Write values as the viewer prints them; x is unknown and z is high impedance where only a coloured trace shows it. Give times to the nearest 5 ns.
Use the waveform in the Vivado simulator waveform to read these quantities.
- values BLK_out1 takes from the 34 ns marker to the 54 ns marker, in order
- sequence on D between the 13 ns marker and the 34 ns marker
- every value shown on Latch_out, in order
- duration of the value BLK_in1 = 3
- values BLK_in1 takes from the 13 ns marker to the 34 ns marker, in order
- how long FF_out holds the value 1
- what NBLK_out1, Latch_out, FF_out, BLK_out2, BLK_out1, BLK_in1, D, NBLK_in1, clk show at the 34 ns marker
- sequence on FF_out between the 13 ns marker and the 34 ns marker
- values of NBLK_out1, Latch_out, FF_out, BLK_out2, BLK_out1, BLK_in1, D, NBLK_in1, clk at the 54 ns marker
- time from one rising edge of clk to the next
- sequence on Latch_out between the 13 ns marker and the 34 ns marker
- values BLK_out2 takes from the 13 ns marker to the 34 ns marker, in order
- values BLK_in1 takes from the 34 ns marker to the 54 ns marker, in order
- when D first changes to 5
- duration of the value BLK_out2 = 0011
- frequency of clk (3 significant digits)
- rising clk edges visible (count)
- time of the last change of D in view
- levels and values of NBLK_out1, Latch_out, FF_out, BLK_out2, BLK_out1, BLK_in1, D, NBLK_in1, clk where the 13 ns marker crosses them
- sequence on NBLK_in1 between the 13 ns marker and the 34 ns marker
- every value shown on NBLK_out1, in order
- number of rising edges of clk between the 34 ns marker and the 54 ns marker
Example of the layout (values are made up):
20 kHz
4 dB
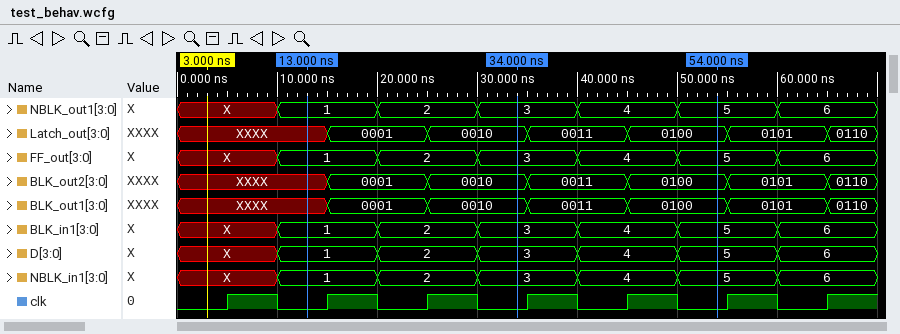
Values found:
0010, 0011, 0100
1, 2, 3
XXXX, 0001, 0010, 0011, 0100, 0101, 0110
10 ns
1, 2, 3
10 ns
NBLK_out1=3, Latch_out=0010, FF_out=3, BLK_out2=0010, BLK_out1=0010, BLK_in1=3, D=3, NBLK_in1=3, clk=0
1, 2, 3
NBLK_out1=5, Latch_out=0100, FF_out=5, BLK_out2=0100, BLK_out1=0100, BLK_in1=5, D=5, NBLK_in1=5, clk=0
10 ns
XXXX, 0001, 0010
XXXX, 0001, 0010
3, 4, 5
50 ns
10 ns
100 MHz
7
60 ns
NBLK_out1=1, Latch_out=XXXX, FF_out=1, BLK_out2=XXXX, BLK_out1=XXXX, BLK_in1=1, D=1, NBLK_in1=1, clk=0
1, 2, 3
X, 1, 2, 3, 4, 5, 6
2
